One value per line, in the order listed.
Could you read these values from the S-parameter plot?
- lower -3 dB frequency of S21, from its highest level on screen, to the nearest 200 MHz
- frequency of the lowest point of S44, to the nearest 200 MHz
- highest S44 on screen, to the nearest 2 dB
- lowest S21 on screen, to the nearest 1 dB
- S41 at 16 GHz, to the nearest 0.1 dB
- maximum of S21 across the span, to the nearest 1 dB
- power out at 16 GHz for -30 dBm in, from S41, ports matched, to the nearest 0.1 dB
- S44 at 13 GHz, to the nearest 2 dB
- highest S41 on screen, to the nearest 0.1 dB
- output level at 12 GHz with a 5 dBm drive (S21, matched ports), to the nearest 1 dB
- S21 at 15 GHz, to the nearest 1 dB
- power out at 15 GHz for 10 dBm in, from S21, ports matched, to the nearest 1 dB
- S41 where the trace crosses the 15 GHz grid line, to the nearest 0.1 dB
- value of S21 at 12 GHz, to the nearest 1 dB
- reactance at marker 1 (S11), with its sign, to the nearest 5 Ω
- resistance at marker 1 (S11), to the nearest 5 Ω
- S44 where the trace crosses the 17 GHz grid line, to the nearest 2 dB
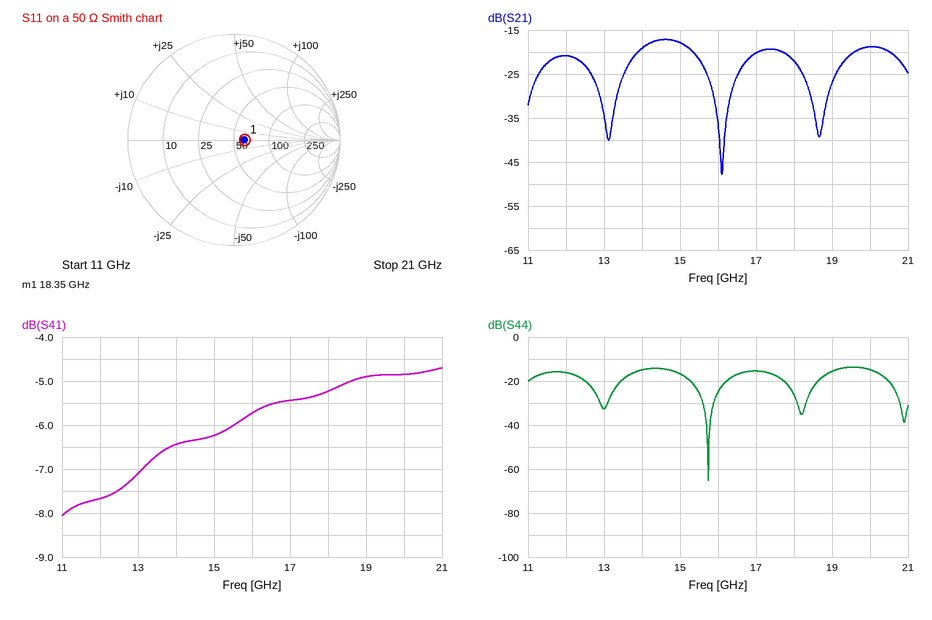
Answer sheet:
13.8 GHz
15.8 GHz
-14 dB
-48 dB
-5.7 dB
-17 dB
-35.7 dBm
-32 dB
-4.7 dB
-16 dBm
-18 dB
-8 dBm
-6.2 dB
-21 dB
0 Ω
60 Ω
-16 dB
